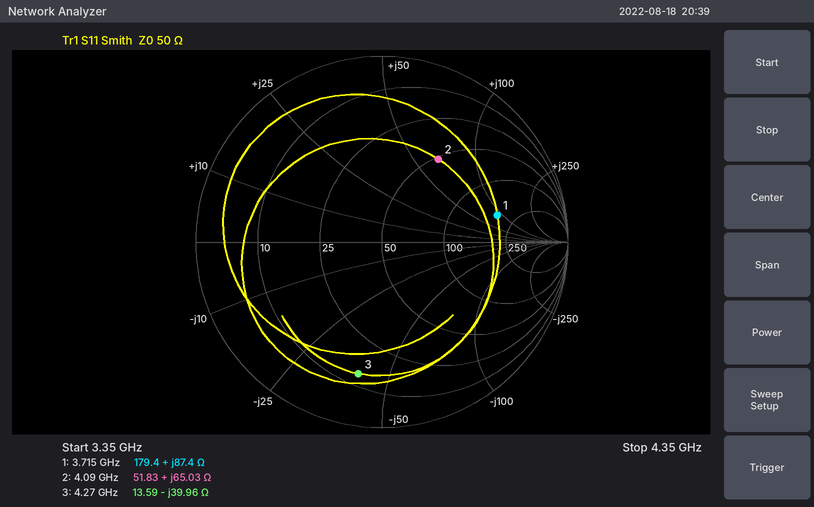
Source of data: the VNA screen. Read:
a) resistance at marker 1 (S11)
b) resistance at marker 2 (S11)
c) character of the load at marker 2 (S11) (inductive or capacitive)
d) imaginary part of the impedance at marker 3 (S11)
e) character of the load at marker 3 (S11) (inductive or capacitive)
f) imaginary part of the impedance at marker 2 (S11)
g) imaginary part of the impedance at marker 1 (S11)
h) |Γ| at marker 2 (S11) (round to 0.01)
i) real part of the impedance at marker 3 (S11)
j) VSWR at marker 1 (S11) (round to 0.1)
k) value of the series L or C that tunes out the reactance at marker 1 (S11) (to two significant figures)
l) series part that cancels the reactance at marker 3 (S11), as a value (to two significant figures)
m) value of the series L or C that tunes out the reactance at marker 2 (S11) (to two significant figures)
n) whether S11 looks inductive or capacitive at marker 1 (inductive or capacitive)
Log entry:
179.4 Ω
51.83 Ω
inductive
-39.96 Ω
capacitive
+65.03 Ω
+87.4 Ω
0.54
13.59 Ω
4.5
490 fF
1.5 nH
600 fF
inductive
